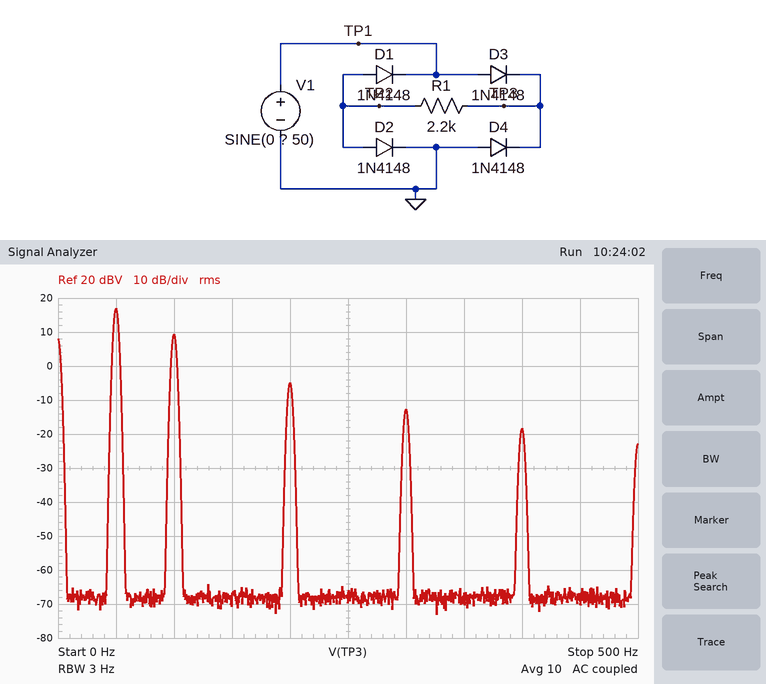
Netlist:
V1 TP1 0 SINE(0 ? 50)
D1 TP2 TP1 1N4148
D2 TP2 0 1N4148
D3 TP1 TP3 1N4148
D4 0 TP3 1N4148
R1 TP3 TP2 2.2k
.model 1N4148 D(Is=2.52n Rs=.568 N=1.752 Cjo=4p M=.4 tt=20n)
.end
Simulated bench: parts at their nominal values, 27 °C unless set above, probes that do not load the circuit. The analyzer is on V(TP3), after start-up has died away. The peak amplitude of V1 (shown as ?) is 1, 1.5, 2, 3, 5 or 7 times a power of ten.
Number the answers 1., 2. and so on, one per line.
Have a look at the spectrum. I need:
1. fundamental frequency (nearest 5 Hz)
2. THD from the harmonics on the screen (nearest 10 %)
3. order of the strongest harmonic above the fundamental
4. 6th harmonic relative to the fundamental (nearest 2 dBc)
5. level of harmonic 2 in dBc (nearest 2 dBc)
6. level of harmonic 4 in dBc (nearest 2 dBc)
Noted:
1. 50 Hz
2. 40 %
3. 2
4. -30 dBc
5. -8 dBc
6. -22 dBc
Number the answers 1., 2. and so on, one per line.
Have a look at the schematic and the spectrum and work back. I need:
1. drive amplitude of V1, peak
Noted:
1. 20 V
